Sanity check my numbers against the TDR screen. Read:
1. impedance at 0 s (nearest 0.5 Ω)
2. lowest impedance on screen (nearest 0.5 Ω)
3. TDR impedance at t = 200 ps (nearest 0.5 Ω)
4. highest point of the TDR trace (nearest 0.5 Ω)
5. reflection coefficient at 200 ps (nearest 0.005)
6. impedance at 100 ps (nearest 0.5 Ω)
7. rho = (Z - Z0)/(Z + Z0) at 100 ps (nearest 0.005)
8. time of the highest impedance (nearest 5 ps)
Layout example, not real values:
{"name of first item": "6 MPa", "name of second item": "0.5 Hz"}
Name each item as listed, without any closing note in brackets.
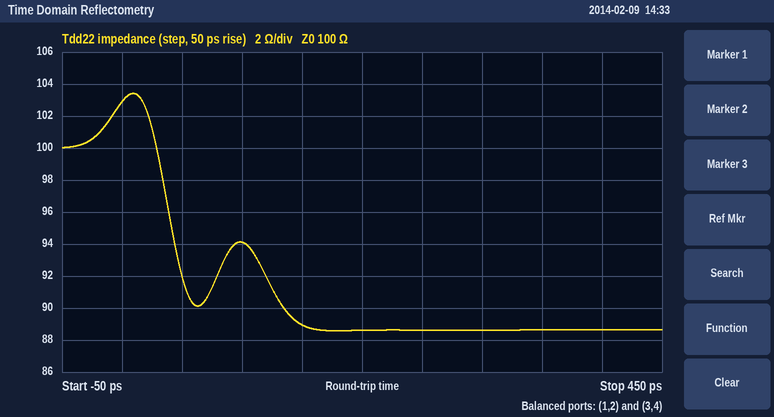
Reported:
{"impedance at 0 s": "103.0 Ω", "lowest impedance on screen": "88.5 Ω", "TDR impedance at t = 200 ps": "88.5 Ω", "highest point of the TDR trace": "103.5 Ω", "reflection coefficient at 200 ps": "-0.060", "impedance at 100 ps": "94.0 Ω", "rho = (Z - Z0)/(Z + Z0) at 100 ps": "-0.030", "time of the highest impedance": "10 ps"}
